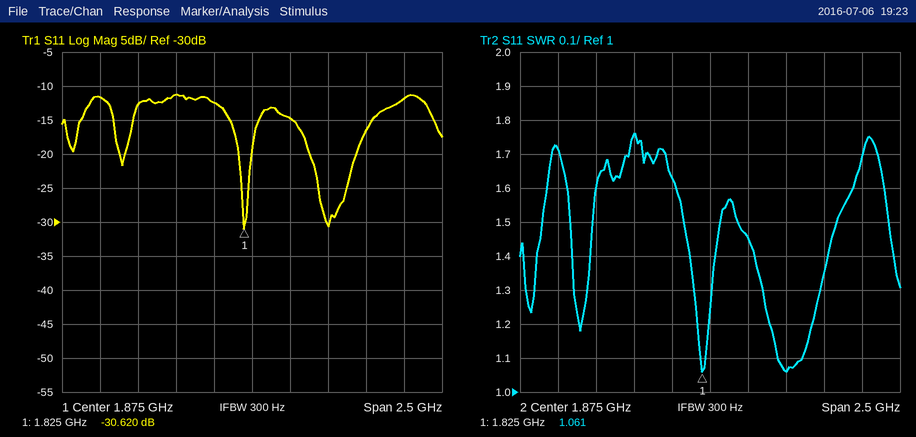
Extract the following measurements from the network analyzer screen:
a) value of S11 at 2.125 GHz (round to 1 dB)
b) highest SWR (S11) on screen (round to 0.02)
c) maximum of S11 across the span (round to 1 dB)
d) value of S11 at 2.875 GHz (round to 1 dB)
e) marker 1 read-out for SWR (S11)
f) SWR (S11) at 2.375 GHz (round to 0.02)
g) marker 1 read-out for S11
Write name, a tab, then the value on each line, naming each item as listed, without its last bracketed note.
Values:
value of S11 at 2.125 GHz	-15 dB
highest SWR (S11) on screen	1.76
maximum of S11 across the span	-11 dB
value of S11 at 2.875 GHz	-12 dB
marker 1 read-out for SWR	1.061
SWR (S11) at 2.375 GHz	1.06
marker 1 read-out for S11	-30.620 dB
